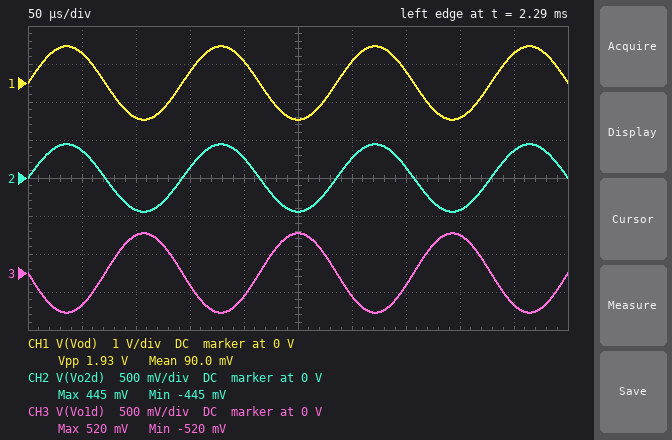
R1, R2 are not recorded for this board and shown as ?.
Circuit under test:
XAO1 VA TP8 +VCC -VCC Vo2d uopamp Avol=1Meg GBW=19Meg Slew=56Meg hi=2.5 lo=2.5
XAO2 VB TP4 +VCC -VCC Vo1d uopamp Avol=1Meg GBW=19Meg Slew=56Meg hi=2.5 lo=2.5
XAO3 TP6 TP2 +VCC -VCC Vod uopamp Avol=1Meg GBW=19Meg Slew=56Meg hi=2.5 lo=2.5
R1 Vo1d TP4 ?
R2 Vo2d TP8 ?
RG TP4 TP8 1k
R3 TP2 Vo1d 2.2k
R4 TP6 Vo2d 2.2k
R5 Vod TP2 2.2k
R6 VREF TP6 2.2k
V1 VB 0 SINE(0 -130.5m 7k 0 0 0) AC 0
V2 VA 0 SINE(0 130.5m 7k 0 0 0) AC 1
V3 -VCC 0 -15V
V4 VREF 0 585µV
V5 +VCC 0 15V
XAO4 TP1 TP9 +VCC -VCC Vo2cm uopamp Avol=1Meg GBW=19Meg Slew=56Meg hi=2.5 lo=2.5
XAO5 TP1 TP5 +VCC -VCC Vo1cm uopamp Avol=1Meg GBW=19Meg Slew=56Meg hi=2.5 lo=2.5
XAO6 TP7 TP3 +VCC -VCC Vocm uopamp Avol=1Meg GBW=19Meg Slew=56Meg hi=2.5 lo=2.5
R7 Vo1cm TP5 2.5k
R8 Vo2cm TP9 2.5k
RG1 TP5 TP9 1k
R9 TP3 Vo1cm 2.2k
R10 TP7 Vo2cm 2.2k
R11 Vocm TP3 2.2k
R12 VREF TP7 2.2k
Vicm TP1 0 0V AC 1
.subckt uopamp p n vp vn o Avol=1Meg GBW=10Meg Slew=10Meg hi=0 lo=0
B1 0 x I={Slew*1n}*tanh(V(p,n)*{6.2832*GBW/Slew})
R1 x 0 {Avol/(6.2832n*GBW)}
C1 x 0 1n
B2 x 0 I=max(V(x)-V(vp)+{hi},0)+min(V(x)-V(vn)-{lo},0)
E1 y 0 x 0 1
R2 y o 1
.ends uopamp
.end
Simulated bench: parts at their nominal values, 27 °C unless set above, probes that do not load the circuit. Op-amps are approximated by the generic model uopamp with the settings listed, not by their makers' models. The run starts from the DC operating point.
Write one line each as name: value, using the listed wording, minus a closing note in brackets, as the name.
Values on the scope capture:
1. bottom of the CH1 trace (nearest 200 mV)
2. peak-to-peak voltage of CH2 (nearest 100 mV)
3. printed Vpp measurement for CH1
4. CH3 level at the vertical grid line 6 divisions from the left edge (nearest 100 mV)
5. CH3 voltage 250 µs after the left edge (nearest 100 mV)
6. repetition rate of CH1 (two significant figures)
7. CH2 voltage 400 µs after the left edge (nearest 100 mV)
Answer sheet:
bottom of the CH1 trace: -1.0 V
peak-to-peak voltage of CH2: 900 mV
printed Vpp measurement for CH1: 1.93 V
CH3 level at the vertical grid line 6 divisions from the left edge: -300 mV
CH3 voltage 250 µs after the left edge: 500 mV
repetition rate of CH1: 7.0 kHz
CH2 voltage 400 µs after the left edge: -400 mV
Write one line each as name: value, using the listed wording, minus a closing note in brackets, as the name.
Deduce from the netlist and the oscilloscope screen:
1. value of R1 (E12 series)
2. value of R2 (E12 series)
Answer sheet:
value of R1: 1.5 kΩ
value of R2: 1.2 kΩ
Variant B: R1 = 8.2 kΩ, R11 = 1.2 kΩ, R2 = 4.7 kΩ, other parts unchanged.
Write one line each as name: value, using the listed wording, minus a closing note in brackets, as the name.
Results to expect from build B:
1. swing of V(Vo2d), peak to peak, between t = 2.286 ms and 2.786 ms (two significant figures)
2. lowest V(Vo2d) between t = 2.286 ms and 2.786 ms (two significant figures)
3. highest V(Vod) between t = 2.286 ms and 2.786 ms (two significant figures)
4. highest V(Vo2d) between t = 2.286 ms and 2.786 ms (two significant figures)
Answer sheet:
swing of V(Vo2d), peak to peak, between t = 2.286 ms and 2.786 ms: 2.7 V
lowest V(Vo2d) between t = 2.286 ms and 2.786 ms: -1.4 V
highest V(Vod) between t = 2.286 ms and 2.786 ms: 3.6 V
highest V(Vo2d) between t = 2.286 ms and 2.786 ms: 1.4 V
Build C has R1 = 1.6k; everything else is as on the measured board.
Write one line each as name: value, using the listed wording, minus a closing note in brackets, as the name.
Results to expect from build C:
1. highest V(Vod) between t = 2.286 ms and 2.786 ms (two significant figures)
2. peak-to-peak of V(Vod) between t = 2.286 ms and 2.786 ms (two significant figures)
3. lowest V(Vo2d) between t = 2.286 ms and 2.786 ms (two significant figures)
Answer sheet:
highest V(Vod) between t = 2.286 ms and 2.786 ms: 990 mV
peak-to-peak of V(Vod) between t = 2.286 ms and 2.786 ms: 2.0 V
lowest V(Vo2d) between t = 2.286 ms and 2.786 ms: -440 mV
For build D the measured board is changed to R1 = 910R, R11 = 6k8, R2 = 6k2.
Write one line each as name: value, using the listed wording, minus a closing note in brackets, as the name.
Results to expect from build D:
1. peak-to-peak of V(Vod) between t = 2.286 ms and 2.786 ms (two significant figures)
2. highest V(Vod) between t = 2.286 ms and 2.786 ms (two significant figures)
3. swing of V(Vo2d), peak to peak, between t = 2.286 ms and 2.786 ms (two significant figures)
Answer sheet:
peak-to-peak of V(Vod) between t = 2.286 ms and 2.786 ms: 4.2 V
highest V(Vod) between t = 2.286 ms and 2.786 ms: 2.1 V
swing of V(Vo2d), peak to peak, between t = 2.286 ms and 2.786 ms: 3.5 V
